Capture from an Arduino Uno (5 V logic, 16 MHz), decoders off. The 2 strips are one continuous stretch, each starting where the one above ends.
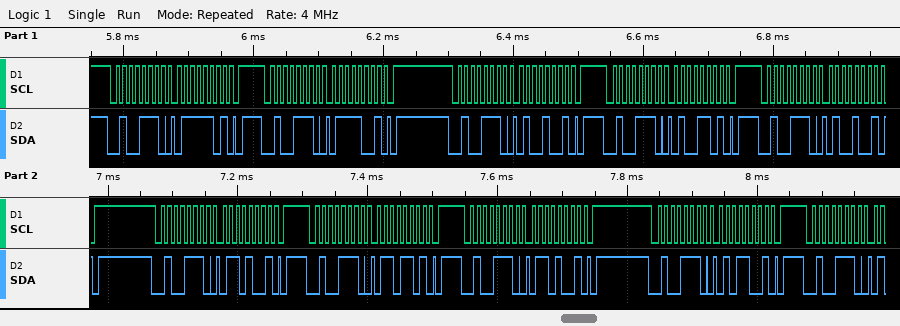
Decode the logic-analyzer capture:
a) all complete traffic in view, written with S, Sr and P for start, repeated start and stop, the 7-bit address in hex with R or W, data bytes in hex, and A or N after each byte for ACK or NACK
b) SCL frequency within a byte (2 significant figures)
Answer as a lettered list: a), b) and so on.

a) S 27W A 7D A P S 27W A 79 A P S 27W A 49 A P S 27W A 4D A P S 27W A 49 A P S 27W A 69 A P S 27W A 6D A P S 27W A 69 A P S 27W A 59 A P S 27W A
b) 100 kHz
